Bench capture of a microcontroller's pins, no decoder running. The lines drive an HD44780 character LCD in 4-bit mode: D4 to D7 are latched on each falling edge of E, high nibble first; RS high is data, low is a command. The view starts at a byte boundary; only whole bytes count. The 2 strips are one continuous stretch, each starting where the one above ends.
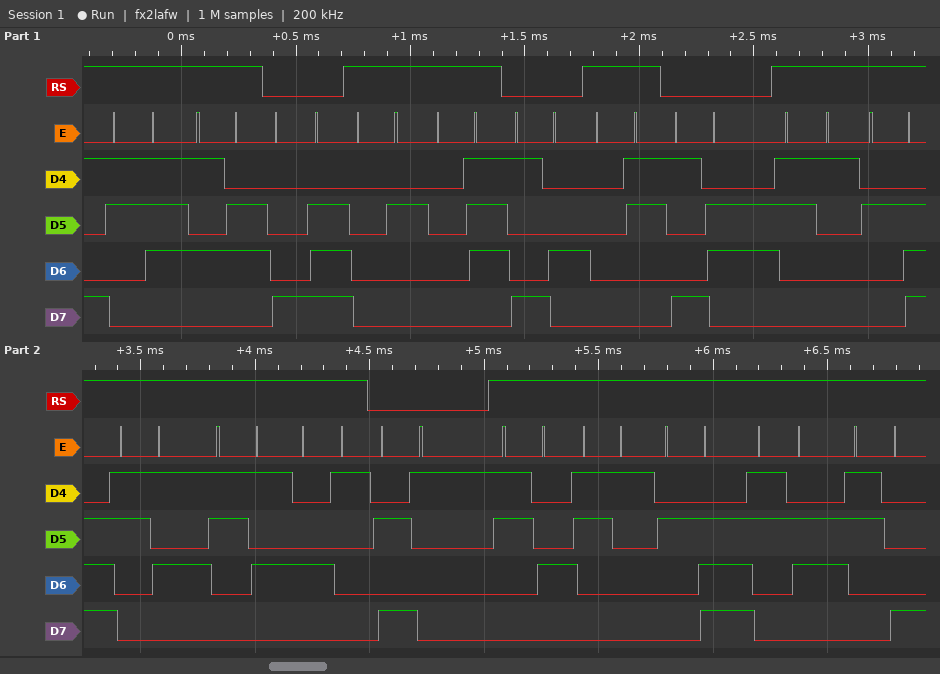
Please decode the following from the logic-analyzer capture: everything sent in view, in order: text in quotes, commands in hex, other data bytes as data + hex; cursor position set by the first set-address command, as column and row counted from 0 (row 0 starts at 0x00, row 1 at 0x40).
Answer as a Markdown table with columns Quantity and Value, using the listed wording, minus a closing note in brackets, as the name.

| Quantity | Value |
|---|---|
| everything sent in view, in order: text in quotes, commands in hex, other data bytes as data + hex | "7V" 0x8E data 02 07 0x94 data 03 0x96 "1.55A" 0xA1 "41.68" |
| cursor position set by the first set-address command, as column and row counted from 0 | column 14, row 0 |
